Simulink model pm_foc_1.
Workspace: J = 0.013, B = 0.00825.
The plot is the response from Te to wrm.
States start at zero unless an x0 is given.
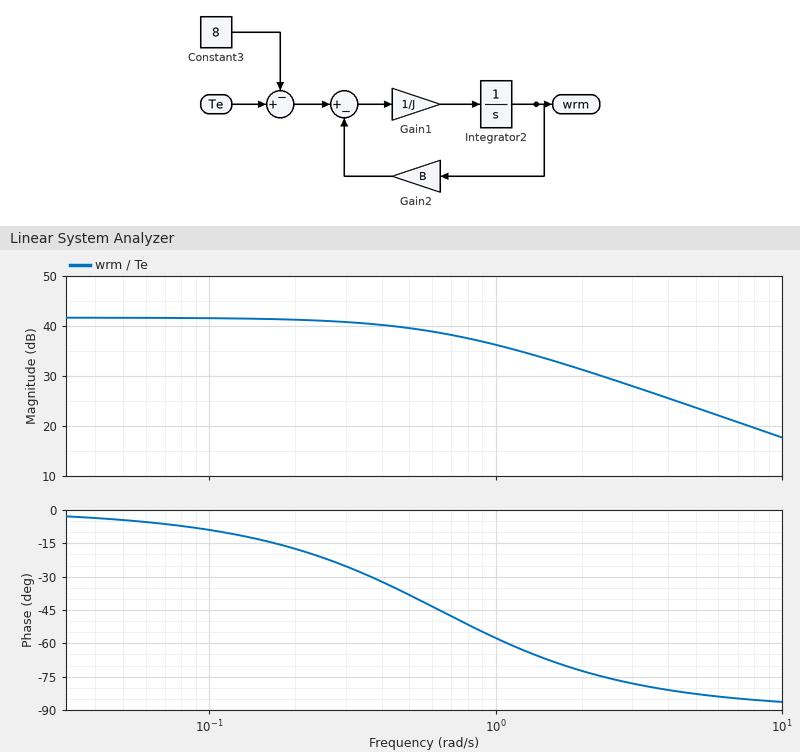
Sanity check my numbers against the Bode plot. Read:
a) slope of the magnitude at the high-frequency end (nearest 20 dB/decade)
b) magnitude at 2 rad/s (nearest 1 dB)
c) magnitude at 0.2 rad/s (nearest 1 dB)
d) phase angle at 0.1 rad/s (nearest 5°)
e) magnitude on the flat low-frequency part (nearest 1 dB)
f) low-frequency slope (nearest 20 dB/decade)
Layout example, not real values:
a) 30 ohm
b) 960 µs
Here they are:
a) -20 dB/decade
b) 31 dB
c) 41 dB
d) -10°
e) 42 dB
f) 0 dB/decade
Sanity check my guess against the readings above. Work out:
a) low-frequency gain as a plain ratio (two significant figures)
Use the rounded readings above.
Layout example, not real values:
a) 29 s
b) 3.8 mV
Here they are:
a) 130
